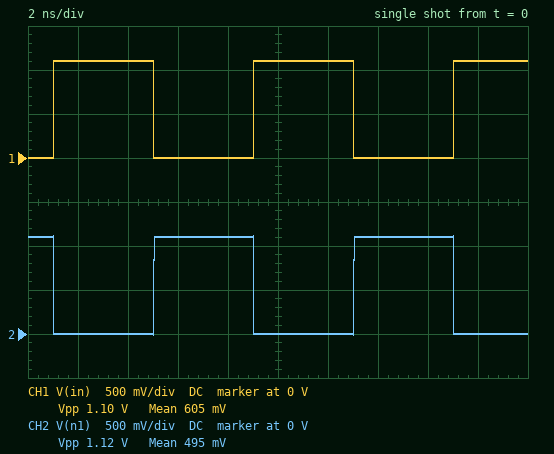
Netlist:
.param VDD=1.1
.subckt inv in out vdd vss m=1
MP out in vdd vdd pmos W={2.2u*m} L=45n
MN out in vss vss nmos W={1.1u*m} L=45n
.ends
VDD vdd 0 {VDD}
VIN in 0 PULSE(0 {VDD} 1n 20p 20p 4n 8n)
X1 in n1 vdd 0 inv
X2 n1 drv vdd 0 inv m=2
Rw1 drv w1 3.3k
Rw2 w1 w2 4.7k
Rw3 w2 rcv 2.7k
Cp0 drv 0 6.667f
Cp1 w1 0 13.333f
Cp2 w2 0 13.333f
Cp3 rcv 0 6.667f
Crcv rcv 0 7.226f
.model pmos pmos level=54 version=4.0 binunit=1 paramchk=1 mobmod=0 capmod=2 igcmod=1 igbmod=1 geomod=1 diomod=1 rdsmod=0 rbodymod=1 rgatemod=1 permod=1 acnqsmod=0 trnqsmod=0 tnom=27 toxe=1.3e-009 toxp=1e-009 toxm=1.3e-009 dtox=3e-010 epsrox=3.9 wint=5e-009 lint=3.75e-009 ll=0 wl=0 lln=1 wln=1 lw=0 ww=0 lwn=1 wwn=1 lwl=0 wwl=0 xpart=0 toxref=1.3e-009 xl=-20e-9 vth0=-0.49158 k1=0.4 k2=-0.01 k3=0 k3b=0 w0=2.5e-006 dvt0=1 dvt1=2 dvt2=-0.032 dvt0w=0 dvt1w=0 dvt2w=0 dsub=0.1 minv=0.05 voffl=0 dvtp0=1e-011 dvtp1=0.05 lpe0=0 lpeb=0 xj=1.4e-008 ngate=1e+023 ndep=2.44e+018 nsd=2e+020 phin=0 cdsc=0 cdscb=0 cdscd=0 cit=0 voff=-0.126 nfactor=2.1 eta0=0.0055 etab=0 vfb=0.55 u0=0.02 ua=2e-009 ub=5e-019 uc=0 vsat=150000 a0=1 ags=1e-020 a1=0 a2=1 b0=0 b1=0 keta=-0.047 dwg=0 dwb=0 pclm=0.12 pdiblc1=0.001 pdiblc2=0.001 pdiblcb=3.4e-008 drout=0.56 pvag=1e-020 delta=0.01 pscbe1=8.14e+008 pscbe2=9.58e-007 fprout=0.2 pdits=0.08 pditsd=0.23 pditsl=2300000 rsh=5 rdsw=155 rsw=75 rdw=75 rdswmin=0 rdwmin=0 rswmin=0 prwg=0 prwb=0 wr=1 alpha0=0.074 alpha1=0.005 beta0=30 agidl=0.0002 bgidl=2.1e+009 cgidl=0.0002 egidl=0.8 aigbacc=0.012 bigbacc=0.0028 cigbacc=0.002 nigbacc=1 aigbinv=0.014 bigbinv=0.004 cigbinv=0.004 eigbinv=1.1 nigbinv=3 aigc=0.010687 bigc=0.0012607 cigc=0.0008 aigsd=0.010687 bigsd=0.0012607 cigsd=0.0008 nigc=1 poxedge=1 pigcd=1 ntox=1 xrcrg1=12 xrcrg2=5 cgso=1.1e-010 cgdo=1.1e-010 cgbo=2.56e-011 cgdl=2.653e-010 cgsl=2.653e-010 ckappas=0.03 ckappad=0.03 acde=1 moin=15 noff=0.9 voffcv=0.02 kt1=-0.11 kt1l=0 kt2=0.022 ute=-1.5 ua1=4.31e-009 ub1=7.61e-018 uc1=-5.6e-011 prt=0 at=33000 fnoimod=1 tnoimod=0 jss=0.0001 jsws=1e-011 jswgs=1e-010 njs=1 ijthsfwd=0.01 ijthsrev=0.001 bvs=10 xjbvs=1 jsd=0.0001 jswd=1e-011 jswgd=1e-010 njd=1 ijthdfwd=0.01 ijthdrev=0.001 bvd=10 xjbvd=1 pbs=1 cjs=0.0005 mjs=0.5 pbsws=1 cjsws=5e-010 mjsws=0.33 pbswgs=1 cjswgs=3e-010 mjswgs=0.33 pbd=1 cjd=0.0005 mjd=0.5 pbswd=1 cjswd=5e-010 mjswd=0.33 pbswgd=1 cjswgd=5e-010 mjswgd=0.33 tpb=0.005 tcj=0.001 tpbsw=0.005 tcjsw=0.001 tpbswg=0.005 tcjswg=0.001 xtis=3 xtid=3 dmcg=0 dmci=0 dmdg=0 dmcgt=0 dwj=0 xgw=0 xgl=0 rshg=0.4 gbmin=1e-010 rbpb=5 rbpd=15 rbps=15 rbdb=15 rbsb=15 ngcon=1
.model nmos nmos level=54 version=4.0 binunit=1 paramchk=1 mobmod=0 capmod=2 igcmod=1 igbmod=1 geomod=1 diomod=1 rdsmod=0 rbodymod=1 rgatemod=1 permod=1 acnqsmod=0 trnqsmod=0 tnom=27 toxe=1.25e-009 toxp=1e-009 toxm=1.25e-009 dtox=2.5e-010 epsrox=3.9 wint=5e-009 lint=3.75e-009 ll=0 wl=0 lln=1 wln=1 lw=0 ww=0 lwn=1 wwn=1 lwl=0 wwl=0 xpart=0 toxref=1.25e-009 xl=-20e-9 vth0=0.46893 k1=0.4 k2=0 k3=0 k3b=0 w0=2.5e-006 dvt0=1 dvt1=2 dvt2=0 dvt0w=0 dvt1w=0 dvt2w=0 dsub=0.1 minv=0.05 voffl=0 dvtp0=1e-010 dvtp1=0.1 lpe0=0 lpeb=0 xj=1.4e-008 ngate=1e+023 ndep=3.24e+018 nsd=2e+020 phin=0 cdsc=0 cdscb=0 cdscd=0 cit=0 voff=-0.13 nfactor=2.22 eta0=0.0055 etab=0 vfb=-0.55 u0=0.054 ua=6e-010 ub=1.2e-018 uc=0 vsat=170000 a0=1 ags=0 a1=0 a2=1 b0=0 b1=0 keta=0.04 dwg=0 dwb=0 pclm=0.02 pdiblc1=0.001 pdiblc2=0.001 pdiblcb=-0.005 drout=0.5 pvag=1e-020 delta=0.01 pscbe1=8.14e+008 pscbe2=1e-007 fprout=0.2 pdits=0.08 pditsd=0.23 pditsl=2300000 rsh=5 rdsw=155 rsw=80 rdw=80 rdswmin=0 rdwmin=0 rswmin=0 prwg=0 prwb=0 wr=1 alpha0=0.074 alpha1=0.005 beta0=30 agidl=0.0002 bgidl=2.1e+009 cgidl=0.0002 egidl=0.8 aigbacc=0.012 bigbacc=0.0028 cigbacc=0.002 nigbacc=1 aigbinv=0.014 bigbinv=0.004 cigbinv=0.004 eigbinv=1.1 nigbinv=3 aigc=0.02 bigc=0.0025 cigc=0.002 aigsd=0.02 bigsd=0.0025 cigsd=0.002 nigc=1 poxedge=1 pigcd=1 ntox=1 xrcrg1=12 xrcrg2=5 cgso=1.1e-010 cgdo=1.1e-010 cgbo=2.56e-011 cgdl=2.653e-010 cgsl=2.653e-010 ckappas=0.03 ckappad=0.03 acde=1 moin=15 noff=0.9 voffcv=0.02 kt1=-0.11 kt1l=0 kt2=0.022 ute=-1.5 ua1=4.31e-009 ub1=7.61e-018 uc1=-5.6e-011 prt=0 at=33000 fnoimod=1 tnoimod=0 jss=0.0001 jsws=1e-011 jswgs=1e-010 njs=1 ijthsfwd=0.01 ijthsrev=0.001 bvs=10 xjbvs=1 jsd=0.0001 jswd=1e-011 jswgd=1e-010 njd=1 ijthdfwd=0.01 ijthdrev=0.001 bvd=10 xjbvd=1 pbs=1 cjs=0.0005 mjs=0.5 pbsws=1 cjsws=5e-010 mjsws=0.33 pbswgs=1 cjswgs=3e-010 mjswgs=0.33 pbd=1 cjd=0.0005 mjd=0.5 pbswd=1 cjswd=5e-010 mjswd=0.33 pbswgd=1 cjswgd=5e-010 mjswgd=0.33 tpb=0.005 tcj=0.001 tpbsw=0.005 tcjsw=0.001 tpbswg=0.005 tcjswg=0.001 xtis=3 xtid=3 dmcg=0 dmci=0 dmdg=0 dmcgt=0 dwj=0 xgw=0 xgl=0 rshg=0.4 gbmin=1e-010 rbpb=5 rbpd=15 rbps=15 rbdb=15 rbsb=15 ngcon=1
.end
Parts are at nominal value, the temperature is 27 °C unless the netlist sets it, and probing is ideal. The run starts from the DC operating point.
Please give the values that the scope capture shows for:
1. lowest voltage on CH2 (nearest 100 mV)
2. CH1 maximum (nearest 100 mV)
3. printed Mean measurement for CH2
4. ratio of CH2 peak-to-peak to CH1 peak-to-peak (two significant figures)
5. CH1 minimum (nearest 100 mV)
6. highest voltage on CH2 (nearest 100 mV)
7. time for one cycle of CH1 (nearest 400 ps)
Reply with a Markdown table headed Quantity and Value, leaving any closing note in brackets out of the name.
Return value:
| Quantity | Value |
|---|---|
| lowest voltage on CH2 | 0 V |
| CH1 maximum | 1.1 V |
| printed Mean measurement for CH2 | 495 mV |
| ratio of CH2 peak-to-peak to CH1 peak-to-peak | 1.0 |
| CH1 minimum | 0 V |
| highest voltage on CH2 | 1.1 V |
| time for one cycle of CH1 | 8.0 ns |
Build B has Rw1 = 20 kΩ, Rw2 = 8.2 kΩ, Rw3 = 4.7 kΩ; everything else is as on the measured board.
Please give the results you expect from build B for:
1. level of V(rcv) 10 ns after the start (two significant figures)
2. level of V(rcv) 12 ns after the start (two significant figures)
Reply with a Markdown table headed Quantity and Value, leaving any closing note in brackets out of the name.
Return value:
| Quantity | Value |
|---|---|
| level of V(rcv) 10 ns after the start | 650 mV |
| level of V(rcv) 12 ns after the start | 1.0 V |
